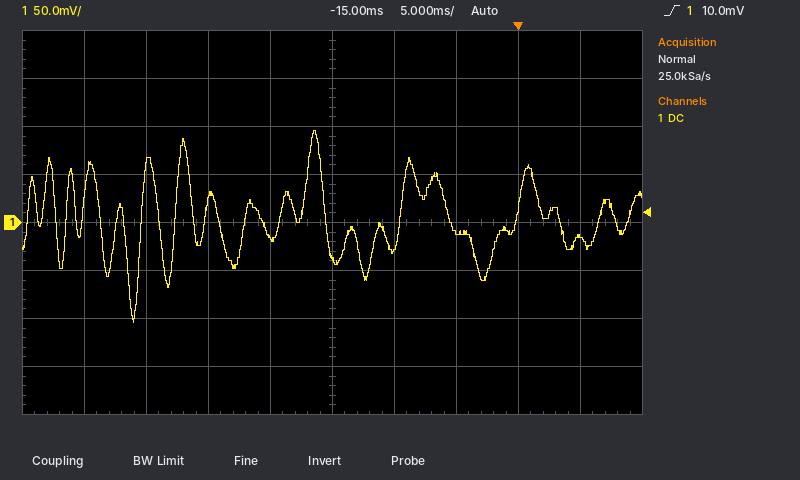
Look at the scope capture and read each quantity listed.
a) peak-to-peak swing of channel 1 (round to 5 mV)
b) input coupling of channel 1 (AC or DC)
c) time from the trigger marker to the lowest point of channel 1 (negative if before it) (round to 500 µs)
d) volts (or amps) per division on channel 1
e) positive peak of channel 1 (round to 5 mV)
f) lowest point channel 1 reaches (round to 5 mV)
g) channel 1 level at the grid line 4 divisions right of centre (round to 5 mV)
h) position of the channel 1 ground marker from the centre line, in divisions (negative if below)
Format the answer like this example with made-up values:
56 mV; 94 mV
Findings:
200 mV; DC; -31.0 ms; 50 mV; 95 mV; -105 mV; -15 mV; 0.0 div
